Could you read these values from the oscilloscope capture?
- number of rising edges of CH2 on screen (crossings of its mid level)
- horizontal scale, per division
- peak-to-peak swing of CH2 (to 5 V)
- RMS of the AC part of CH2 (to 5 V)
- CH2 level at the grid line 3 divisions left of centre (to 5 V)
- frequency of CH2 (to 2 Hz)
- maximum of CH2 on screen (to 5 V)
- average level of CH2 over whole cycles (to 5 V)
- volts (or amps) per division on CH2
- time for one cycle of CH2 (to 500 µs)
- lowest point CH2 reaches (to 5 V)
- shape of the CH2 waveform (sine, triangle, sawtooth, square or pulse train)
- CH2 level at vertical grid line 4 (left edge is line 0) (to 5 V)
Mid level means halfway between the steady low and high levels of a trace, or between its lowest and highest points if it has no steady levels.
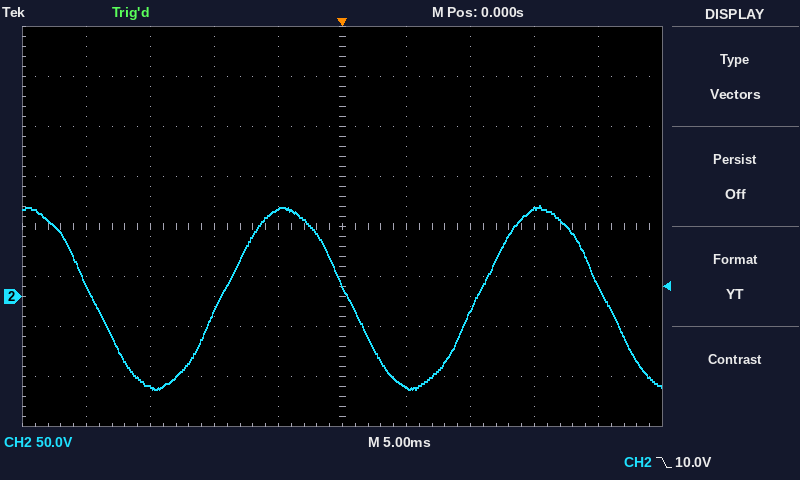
2
5 ms
185 V
65 V
-90 V
50 Hz
90 V
0 V
50 V
20.0 ms
-95 V
sine
85 V
